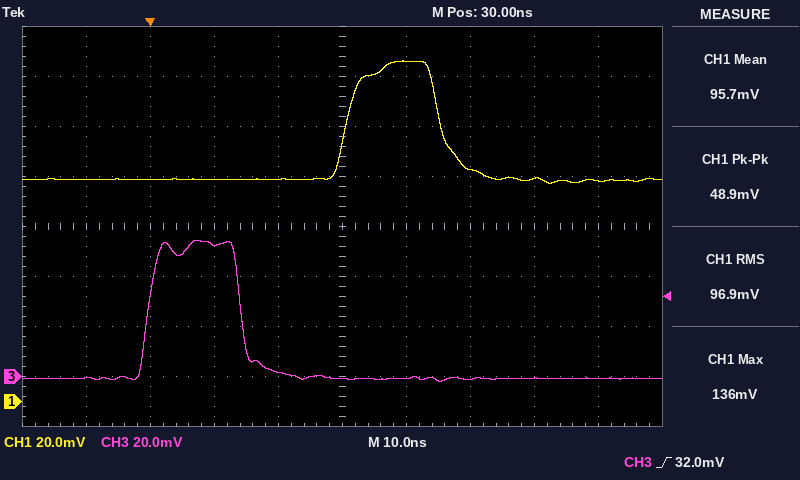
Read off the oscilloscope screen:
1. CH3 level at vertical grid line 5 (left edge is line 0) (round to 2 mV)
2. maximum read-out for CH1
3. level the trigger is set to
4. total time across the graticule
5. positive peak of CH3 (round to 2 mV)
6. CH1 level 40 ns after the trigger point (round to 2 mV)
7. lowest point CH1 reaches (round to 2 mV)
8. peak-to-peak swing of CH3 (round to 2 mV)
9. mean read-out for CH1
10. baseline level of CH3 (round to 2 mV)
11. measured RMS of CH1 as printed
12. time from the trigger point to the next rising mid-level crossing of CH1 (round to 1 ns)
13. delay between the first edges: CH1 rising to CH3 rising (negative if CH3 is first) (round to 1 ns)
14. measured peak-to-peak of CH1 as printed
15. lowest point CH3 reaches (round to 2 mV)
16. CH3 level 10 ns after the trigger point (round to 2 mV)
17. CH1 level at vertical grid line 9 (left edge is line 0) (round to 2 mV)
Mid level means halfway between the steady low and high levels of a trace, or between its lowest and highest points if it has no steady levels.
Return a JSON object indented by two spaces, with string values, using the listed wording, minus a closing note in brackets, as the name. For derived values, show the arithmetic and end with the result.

{
  "CH3 level at vertical grid line 5 (left edge is line 0)": "0 mV",
  "maximum read-out for CH1": "136 mV",
  "level the trigger is set to": "32.0 mV",
  "total time across the graticule": "100 ns",
  "positive peak of CH3": "54 mV",
  "CH1 level 40 ns after the trigger point": "136 mV",
  "lowest point CH1 reaches": "88 mV",
  "peak-to-peak swing of CH3": "54 mV − (-2 mV) = 56 mV",
  "mean read-out for CH1": "95.7 mV",
  "baseline level of CH3": "0 mV",
  "measured RMS of CH1 as printed": "96.9 mV",
  "time from the trigger point to the next rising mid-level crossing of CH1": "31 ns",
  "delay between the first edges: CH1 rising to CH3 rising (negative if CH3 is first)": "-31 ns",
  "measured peak-to-peak of CH1 as printed": "48.9 mV",
  "lowest point CH3 reaches": "-2 mV",
  "CH3 level 10 ns after the trigger point": "52 mV",
  "CH1 level at vertical grid line 9 (left edge is line 0)": "88 mV"
}
